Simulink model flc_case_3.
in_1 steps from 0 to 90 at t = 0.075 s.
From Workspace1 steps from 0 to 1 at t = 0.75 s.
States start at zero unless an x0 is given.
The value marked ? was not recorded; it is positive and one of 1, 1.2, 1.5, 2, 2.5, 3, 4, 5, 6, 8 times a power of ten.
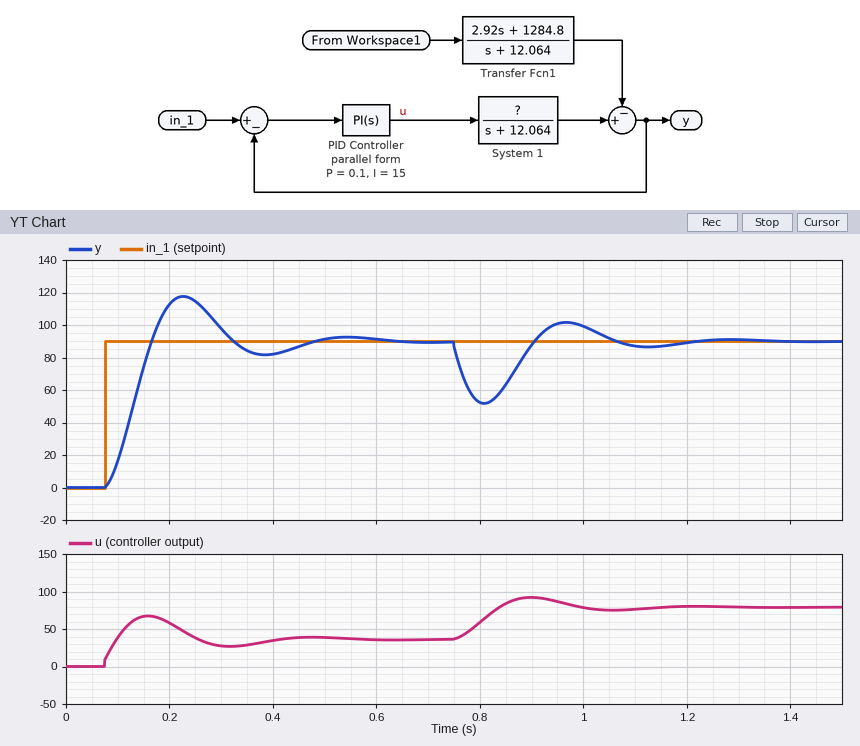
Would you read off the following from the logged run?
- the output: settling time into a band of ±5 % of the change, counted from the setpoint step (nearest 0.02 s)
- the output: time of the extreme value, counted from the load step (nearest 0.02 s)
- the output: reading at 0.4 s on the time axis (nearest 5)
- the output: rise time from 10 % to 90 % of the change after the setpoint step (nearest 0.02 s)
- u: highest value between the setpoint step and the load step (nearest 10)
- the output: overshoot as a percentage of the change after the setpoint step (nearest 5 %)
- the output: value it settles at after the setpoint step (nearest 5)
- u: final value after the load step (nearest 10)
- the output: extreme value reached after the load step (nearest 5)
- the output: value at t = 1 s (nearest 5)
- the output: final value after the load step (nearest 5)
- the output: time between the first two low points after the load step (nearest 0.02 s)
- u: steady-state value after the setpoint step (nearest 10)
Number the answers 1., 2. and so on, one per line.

1. 0.36 s
2. 0.06 s
3. 80
4. 0.06 s
5. 70
6. 30 %
7. 90
8. 80
9. 50
10. 100
11. 90
12. 0.32 s
13. 40
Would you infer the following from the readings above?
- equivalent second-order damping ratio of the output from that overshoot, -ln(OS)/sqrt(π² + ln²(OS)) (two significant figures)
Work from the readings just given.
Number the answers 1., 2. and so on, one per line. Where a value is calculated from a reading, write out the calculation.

1. ln(0.3) = -1.204; 1.204 / sqrt(9.870 + 1.450) = 0.36
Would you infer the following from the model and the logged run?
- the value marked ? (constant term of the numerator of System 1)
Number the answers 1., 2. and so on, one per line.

1. 30
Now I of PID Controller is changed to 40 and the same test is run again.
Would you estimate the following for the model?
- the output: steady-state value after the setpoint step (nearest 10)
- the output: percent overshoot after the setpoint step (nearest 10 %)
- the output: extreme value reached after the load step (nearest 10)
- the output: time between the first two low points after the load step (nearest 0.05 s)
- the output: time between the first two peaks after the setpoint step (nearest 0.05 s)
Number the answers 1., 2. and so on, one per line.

1. 90
2. 50 %
3. 60
4. 0.20 s
5. 0.20 s
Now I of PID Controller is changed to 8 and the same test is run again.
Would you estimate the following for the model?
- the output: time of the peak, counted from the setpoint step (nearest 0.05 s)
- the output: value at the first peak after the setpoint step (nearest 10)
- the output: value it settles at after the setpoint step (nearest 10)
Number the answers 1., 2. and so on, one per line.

1. 0.20 s
2. 110
3. 90
